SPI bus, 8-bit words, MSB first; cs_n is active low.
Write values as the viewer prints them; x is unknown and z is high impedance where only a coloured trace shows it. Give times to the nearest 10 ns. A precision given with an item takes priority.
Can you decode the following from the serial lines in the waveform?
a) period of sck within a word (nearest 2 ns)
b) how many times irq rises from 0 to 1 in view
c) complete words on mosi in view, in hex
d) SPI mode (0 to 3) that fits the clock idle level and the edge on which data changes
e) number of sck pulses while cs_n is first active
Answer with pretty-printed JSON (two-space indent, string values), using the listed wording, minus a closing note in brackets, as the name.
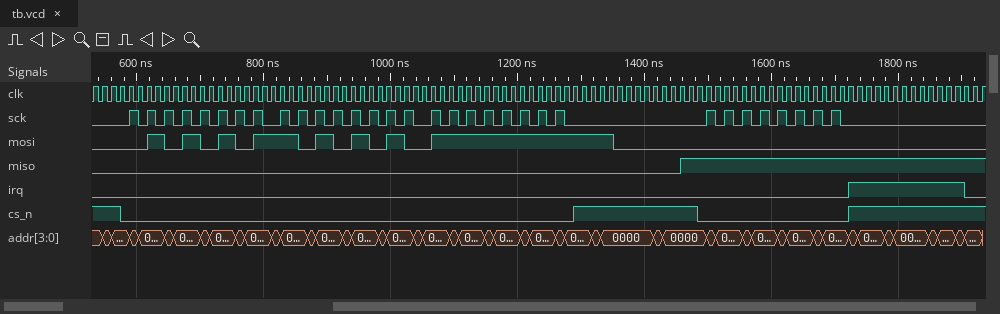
{
  "period of sck within a word": "28 ns",
  "how many times irq rises from 0 to 1 in view": "1",
  "complete words on mosi in view, in hex": "55, AA, FF, 00",
  "SPI mode (0 to 3) that fits the clock idle level and the edge on which data changes": "1",
  "number of sck pulses while cs_n is first active": "24"
}
